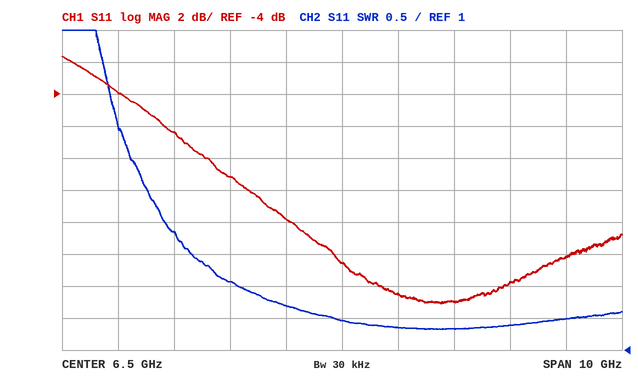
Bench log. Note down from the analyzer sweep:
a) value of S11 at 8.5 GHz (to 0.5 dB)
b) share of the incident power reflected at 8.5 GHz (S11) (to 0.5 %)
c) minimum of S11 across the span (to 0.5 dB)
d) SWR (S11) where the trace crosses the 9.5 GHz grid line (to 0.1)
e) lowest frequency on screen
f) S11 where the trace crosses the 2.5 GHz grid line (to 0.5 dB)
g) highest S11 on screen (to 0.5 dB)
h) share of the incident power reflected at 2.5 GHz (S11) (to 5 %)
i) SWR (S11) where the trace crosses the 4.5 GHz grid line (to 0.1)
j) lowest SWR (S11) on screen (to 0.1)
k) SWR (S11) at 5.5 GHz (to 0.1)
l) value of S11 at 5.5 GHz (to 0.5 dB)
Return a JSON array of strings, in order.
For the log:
["-17.0 dB", "2.0 %", "-17.0 dB", "1.4", "1.5 GHz", "-4.0 dB", "-1.5 dB", "40 %", "2.1", "1.3", "1.7", "-12.0 dB"]
